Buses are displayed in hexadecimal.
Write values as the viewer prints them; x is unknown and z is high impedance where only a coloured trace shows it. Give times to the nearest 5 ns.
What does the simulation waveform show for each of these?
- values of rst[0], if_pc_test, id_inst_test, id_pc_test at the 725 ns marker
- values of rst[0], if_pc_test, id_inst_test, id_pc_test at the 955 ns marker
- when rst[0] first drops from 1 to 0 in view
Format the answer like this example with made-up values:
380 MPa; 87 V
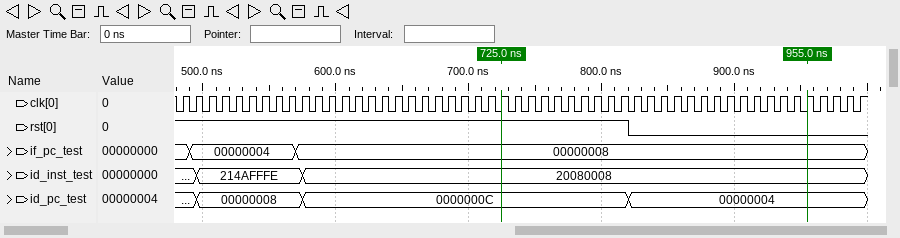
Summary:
rst[0]=1, if_pc_test=00000008, id_inst_test=20080008, id_pc_test=0000000C; rst[0]=0, if_pc_test=00000008, id_inst_test=20080008, id_pc_test=00000004; 820 ns
